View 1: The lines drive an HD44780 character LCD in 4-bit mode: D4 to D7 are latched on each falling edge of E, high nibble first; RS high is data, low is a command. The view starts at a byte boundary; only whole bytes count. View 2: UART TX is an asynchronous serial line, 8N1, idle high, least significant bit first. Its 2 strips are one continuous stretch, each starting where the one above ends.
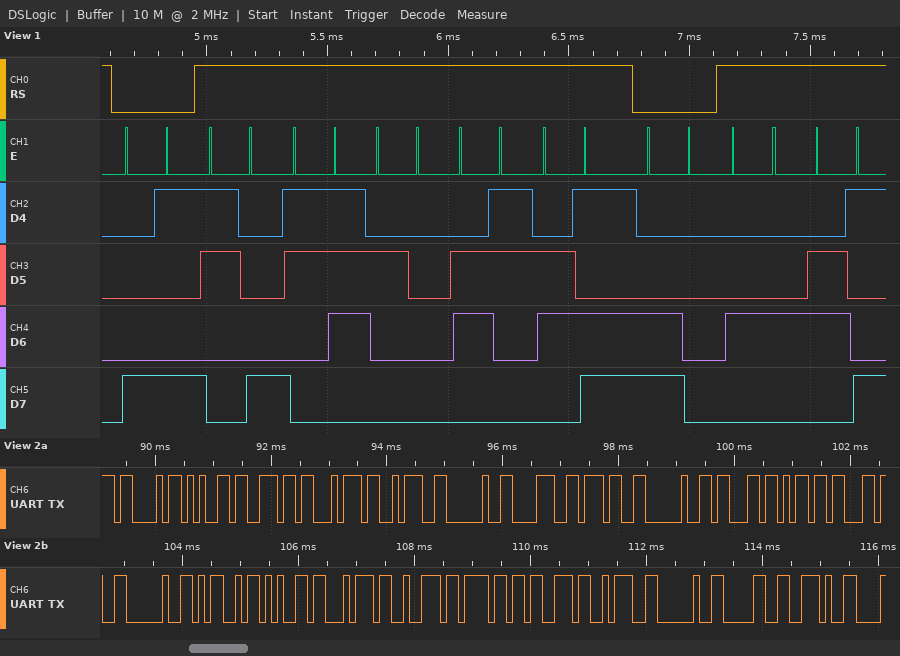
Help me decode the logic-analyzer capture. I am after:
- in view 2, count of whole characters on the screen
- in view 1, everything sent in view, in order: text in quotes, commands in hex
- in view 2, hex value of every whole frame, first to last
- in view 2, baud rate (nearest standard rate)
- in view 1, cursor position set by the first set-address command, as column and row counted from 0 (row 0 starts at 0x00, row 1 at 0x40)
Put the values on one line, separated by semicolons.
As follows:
23; 0x89 "87 cm" 0xC0 "Di"; 43 65 6E 74 3A 20 38 37 20 63 6D 2C 20 4D 65 74 72 6F 73 3A 20 30 2E; 9600 baud; column 9, row 0
